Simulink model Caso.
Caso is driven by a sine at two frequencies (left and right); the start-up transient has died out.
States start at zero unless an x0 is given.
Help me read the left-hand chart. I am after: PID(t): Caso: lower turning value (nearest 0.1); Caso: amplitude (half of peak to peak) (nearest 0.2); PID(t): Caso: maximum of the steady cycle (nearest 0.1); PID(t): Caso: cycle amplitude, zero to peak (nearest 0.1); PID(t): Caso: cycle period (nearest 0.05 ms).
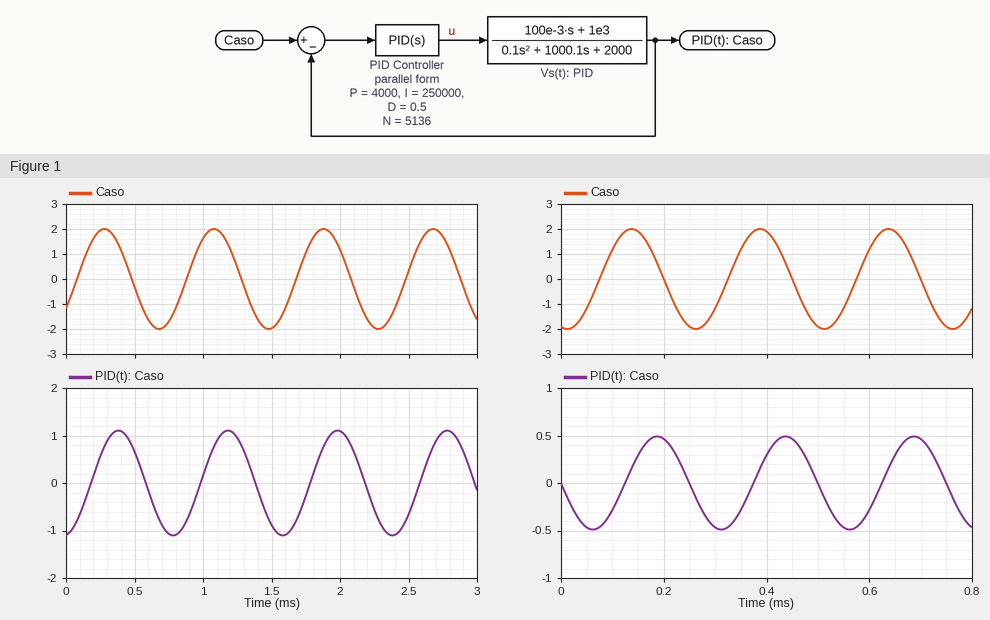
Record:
-1.1
2.0
1.1
1.1
0.80 ms
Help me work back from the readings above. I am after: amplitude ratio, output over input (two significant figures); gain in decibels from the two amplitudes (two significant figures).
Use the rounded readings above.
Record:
0.55
-5.2 dB
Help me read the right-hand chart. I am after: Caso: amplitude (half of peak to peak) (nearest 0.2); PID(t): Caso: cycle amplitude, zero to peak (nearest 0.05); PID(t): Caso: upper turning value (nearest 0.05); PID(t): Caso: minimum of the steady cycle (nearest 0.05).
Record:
2.0
0.50
0.50
-0.50
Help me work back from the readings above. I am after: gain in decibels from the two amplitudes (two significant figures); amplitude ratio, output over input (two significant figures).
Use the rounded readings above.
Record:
-12 dB
0.25
